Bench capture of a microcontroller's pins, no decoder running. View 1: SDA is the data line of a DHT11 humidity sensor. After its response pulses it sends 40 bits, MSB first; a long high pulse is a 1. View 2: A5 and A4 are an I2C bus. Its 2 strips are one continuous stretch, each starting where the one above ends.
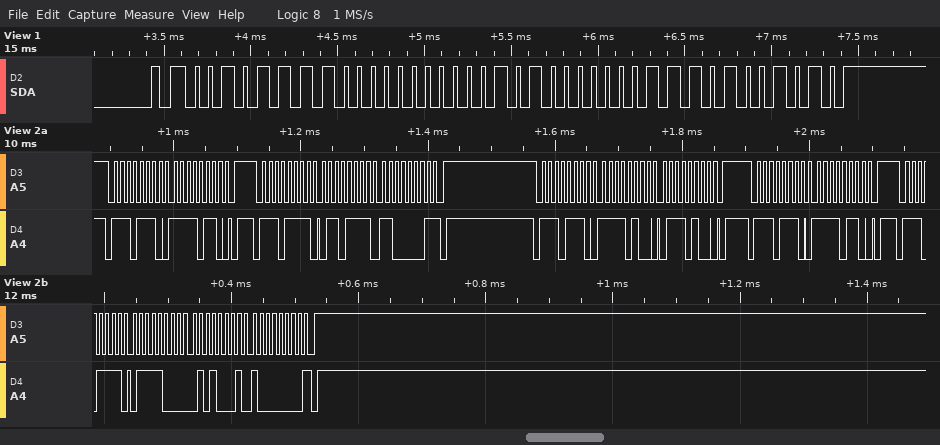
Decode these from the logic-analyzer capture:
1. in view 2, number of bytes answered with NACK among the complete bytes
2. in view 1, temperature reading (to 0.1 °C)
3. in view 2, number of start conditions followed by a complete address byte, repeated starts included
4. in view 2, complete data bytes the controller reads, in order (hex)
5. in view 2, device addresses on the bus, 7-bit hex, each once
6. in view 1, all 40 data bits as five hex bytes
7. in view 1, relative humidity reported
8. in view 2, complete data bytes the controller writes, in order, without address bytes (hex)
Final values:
2
20.7 °C
5
6F C1 78 51 80
0x77
2F 00 14 07 4A
47 %
F6 F4 74 F6
